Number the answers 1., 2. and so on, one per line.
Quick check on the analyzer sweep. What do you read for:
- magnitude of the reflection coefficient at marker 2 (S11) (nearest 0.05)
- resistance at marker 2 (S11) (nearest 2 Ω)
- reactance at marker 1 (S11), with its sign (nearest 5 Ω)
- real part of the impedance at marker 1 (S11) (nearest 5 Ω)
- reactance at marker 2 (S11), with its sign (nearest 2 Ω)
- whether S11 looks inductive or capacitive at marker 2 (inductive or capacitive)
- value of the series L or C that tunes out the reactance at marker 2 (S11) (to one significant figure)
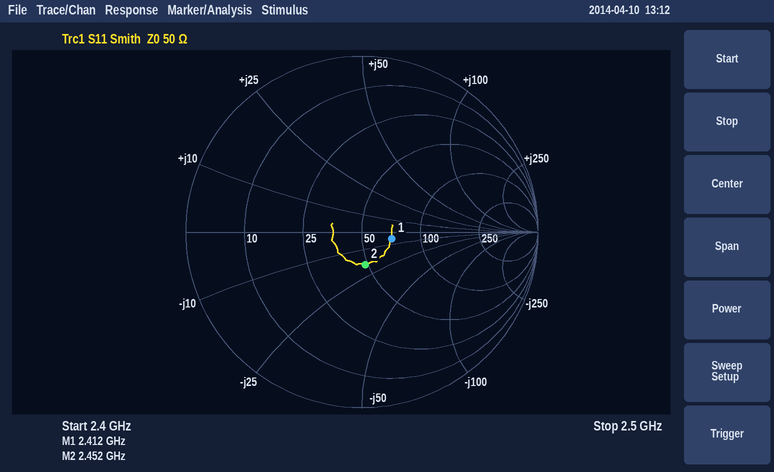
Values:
1. 0.20
2. 48 Ω
3. -5 Ω
4. 70 Ω
5. -18 Ω
6. capacitive
7. 1 nH
